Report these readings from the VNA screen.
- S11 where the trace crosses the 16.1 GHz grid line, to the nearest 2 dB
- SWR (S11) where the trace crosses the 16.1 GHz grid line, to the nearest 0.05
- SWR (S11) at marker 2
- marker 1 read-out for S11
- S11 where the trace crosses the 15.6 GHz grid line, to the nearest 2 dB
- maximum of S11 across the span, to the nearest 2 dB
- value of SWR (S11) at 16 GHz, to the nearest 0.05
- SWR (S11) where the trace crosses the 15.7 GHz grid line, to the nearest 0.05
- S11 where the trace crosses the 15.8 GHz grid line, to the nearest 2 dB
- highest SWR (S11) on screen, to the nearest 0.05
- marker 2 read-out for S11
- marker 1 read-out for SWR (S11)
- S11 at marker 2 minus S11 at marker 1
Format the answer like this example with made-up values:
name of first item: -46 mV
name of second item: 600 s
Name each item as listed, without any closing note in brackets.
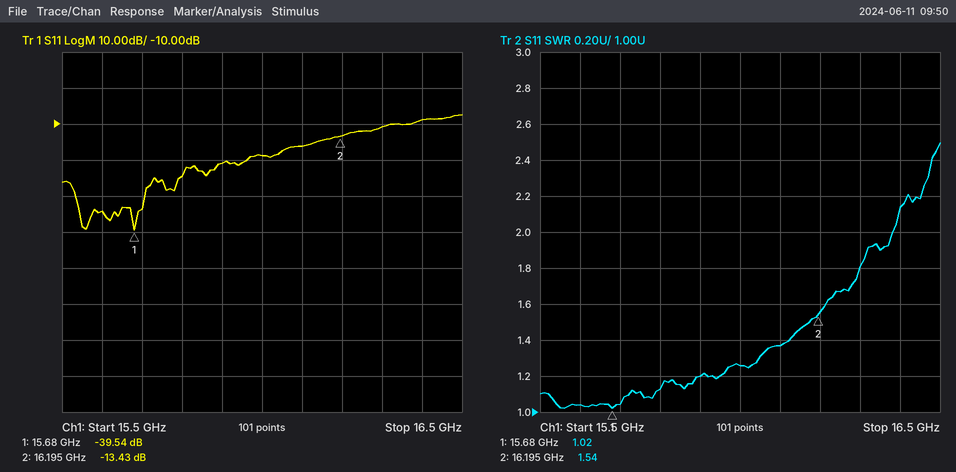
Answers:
S11 where the trace crosses the 16.1 GHz grid line, to the nearest 2 dB: -16 dB
SWR (S11) where the trace crosses the 16.1 GHz grid line, to the nearest 0.05: 1.35
SWR (S11) at marker 2: 1.54
marker 1 read-out for S11: -39.54 dB
S11 where the trace crosses the 15.6 GHz grid line, to the nearest 2 dB: -34 dB
maximum of S11 across the span, to the nearest 2 dB: -8 dB
value of SWR (S11) at 16 GHz, to the nearest 0.05: 1.25
SWR (S11) where the trace crosses the 15.7 GHz grid line, to the nearest 0.05: 1.05
S11 where the trace crosses the 15.8 GHz grid line, to the nearest 2 dB: -24 dB
highest SWR (S11) on screen, to the nearest 0.05: 2.50
marker 2 read-out for S11: -13.43 dB
marker 1 read-out for SWR: 1.02
S11 at marker 2 minus S11 at marker 1: 26.11 dB
